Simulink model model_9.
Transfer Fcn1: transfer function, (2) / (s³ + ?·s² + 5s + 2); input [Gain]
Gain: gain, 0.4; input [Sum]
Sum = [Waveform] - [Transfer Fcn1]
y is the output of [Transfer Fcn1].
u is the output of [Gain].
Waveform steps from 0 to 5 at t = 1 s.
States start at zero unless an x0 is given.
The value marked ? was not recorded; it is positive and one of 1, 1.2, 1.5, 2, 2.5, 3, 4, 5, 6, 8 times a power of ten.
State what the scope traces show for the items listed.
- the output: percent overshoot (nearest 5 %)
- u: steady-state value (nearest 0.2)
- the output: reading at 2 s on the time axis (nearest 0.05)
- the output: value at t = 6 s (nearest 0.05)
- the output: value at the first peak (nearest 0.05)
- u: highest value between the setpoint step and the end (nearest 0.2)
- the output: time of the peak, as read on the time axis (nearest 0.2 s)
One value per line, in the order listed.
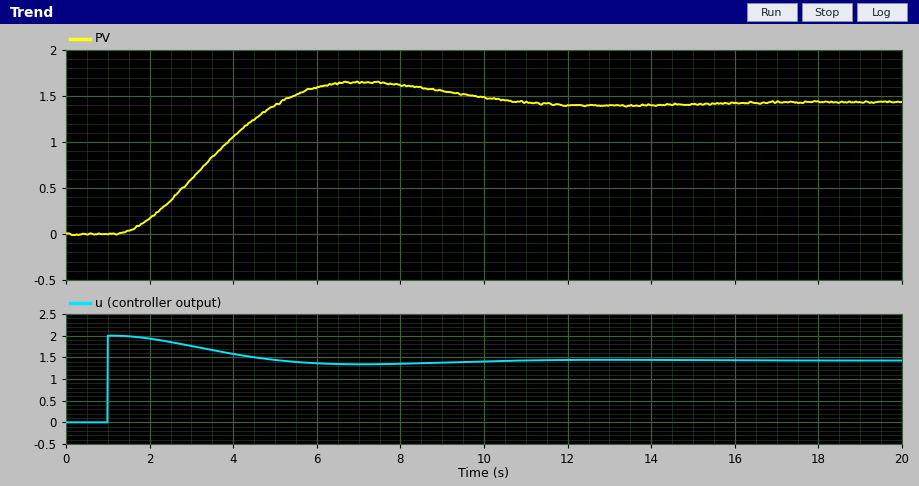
15 %
1.4
0.15
1.60
1.65
2.0
7.0 s
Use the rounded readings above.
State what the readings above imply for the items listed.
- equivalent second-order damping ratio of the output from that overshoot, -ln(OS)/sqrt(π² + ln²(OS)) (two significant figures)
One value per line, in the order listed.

0.52
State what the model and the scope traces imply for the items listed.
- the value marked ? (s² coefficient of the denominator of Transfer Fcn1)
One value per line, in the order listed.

8
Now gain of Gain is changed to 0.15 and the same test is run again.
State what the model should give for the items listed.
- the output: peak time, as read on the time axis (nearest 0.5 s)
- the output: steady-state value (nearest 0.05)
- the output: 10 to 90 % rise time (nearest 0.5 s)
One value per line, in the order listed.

8.0 s
0.65
3.0 s
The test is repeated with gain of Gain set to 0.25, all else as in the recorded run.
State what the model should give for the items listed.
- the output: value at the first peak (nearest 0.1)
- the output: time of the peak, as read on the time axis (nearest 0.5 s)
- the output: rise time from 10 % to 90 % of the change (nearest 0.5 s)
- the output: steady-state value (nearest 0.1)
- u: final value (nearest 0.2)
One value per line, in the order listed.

1.1
7.5 s
3.0 s
1.0
1.0
